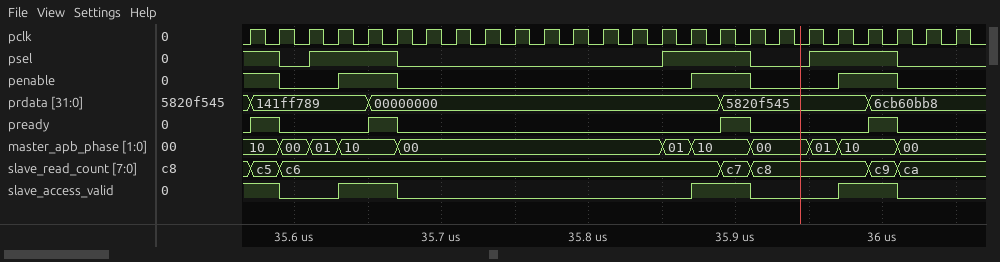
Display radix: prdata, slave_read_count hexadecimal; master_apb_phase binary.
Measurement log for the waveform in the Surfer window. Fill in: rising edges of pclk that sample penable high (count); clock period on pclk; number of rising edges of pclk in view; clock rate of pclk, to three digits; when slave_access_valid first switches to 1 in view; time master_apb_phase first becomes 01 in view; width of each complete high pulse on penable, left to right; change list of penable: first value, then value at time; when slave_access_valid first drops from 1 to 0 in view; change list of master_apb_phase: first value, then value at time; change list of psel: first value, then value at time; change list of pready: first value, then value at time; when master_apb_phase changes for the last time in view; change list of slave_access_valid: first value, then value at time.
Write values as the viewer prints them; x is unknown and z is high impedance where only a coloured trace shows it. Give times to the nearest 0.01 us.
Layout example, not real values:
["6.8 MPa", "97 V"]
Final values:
["8", "0.02 us", "25", "50.0 MHz", "35.63 us", "35.61 us", "0.04 us, 0.04 us, 0.04 us", "1, 0 at 35.59 us, 1 at 35.63 us, 0 at 35.67 us, 1 at 35.87 us, 0 at 35.91 us, 1 at 35.97 us, 0 at 36.01 us", "35.59 us", "10, 00 at 35.59 us, 01 at 35.61 us, 10 at 35.63 us, 00 at 35.67 us, 01 at 35.85 us, 10 at 35.87 us, 00 at 35.91 us, 01 at 35.95 us, 10 at 35.97 us, 00 at 36.01 us", "1, 0 at 35.59 us, 1 at 35.61 us, 0 at 35.67 us, 1 at 35.85 us, 0 at 35.91 us, 1 at 35.95 us, 0 at 36.01 us", "0, 1 at 35.57 us, 0 at 35.59 us, 1 at 35.65 us, 0 at 35.67 us, 1 at 35.89 us, 0 at 35.91 us, 1 at 35.99 us, 0 at 36.01 us", "36.01 us", "1, 0 at 35.59 us, 1 at 35.63 us, 0 at 35.67 us, 1 at 35.87 us, 0 at 35.91 us, 1 at 35.97 us, 0 at 36.01 us"]
